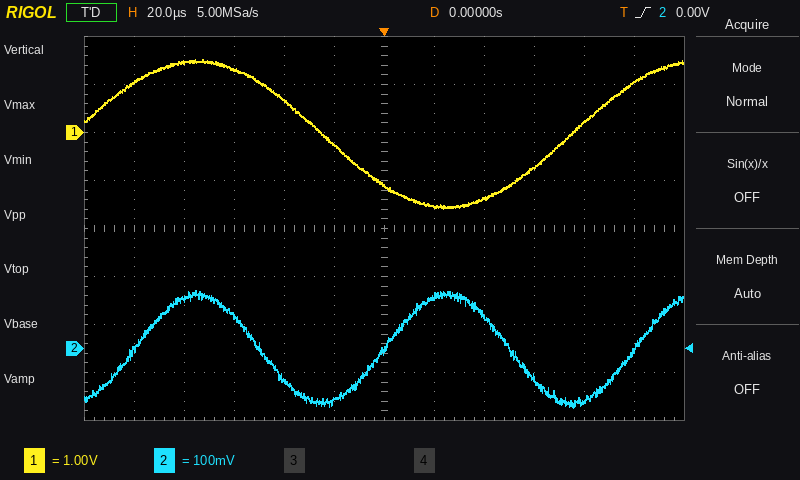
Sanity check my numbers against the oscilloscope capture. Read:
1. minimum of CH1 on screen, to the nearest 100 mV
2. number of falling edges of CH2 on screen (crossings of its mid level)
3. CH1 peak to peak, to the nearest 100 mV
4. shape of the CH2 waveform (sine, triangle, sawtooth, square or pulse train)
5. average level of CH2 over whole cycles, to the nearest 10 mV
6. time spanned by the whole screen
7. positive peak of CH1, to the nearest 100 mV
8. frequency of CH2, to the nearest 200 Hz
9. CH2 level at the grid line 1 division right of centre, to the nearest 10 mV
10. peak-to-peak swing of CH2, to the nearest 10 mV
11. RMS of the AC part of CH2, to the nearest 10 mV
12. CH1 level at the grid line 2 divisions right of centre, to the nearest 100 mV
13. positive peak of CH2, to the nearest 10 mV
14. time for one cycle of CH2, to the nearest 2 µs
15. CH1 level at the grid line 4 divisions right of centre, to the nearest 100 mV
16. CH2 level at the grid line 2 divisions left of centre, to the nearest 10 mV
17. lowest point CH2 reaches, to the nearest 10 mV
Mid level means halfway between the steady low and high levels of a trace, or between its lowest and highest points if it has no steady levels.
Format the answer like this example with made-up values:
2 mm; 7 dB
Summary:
-1.6 V; 2; 3.1 V; sine; 0 mV; 240 µs; 1.5 V; 10.0 kHz; 110 mV; 240 mV; 80 mV; -1.4 V; 120 mV; 100 µs; 200 mV; -60 mV; -120 mV
